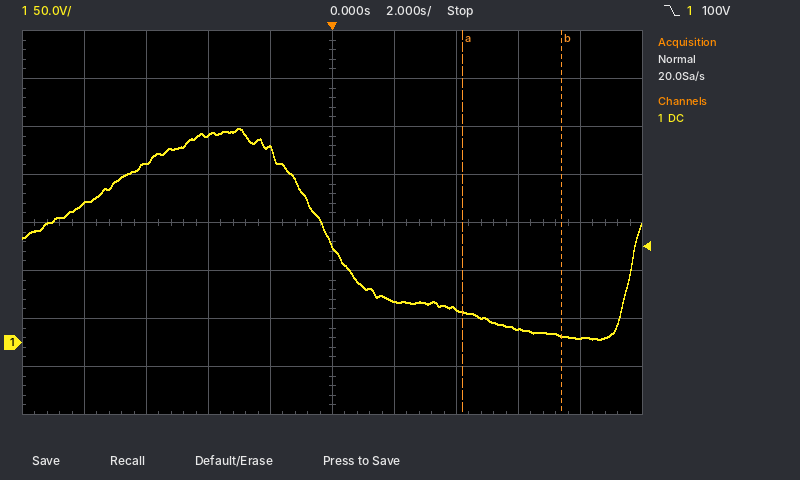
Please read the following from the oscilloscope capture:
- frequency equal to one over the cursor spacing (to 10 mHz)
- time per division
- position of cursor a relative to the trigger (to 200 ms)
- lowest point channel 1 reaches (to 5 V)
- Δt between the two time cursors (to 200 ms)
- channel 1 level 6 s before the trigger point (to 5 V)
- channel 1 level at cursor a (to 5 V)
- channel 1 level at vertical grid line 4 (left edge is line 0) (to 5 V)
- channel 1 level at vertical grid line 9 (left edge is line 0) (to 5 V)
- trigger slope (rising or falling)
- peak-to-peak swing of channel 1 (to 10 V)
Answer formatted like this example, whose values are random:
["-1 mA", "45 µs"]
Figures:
["310 mHz", "2 s", "+4.2 s", "5 V", "3.2 s", "185 V", "30 V", "200 V", "5 V", "falling", "220 V"]
